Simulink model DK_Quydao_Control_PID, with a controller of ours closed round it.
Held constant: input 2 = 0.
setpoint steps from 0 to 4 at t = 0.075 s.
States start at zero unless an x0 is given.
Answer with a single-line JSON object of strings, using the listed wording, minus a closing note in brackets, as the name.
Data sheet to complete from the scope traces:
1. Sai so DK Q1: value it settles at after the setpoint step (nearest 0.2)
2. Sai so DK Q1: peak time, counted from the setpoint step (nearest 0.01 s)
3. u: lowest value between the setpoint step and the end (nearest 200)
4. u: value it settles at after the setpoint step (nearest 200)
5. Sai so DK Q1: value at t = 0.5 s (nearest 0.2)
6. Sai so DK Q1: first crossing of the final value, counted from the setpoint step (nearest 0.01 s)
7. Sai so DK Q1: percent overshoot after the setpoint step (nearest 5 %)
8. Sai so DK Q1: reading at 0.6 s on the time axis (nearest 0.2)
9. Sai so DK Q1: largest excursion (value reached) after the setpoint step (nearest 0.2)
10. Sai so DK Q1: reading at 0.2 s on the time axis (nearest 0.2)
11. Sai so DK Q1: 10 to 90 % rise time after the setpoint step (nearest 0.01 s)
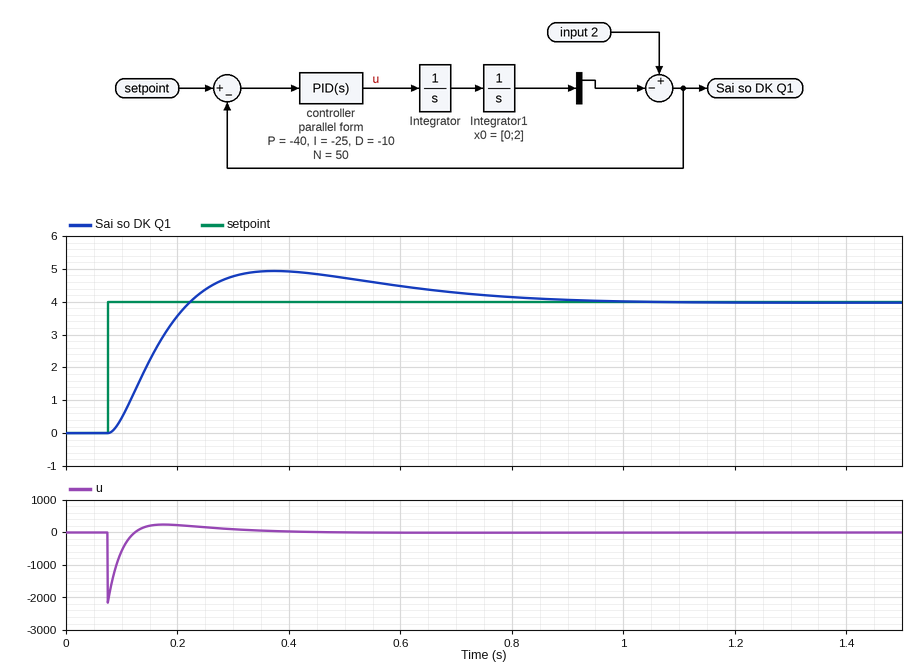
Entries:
{"Sai so DK Q1: value it settles at after the setpoint step": "4.0", "Sai so DK Q1: peak time, counted from the setpoint step": "0.30 s", "u: lowest value between the setpoint step and the end": "-2200", "u: value it settles at after the setpoint step": "0", "Sai so DK Q1: value at t = 0.5 s": "4.8", "Sai so DK Q1: first crossing of the final value, counted from the setpoint step": "0.15 s", "Sai so DK Q1: percent overshoot after the setpoint step": "25 %", "Sai so DK Q1: reading at 0.6 s on the time axis": "4.4", "Sai so DK Q1: largest excursion (value reached) after the setpoint step": "5.0", "Sai so DK Q1: reading at 0.2 s on the time axis": "3.6", "Sai so DK Q1: 10 to 90 % rise time after the setpoint step": "0.10 s"}
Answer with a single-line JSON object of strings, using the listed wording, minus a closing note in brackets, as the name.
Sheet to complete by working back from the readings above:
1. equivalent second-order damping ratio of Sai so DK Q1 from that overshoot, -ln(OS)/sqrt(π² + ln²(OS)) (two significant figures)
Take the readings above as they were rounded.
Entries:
{"equivalent second-order damping ratio of Sai so DK Q1 from that overshoot, -ln(OS)/sqrt(π² + ln²(OS))": "0.40"}
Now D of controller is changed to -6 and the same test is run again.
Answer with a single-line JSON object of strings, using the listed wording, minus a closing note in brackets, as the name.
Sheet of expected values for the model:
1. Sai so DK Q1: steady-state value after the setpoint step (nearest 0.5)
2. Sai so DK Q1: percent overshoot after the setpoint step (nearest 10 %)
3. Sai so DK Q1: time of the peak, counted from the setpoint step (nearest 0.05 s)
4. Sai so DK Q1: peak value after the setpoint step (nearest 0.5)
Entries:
{"Sai so DK Q1: steady-state value after the setpoint step": "4.0", "Sai so DK Q1: percent overshoot after the setpoint step": "40 %", "Sai so DK Q1: time of the peak, counted from the setpoint step": "0.35 s", "Sai so DK Q1: peak value after the setpoint step": "5.5"}
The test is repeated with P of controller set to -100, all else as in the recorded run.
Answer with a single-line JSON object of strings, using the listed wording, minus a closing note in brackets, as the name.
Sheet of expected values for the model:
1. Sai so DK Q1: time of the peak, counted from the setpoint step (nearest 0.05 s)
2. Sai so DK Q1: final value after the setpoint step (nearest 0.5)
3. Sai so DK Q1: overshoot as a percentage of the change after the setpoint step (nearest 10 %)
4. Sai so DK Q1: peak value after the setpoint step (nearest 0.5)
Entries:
{"Sai so DK Q1: time of the peak, counted from the setpoint step": "0.20 s", "Sai so DK Q1: final value after the setpoint step": "4.0", "Sai so DK Q1: overshoot as a percentage of the change after the setpoint step": "40 %", "Sai so DK Q1: peak value after the setpoint step": "5.5"}
